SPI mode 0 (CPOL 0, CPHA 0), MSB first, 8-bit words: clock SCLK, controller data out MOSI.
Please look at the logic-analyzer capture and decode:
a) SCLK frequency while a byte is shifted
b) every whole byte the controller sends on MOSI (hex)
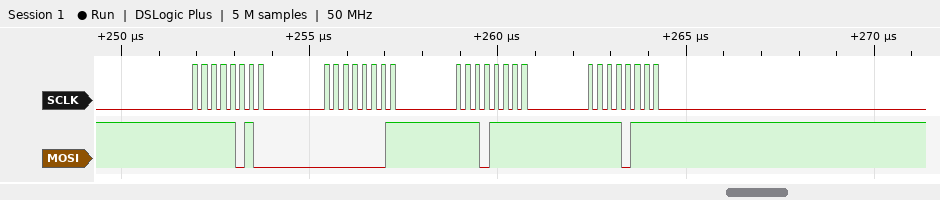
4 MHz
0xFA 0x01 0xEF 0xF7
